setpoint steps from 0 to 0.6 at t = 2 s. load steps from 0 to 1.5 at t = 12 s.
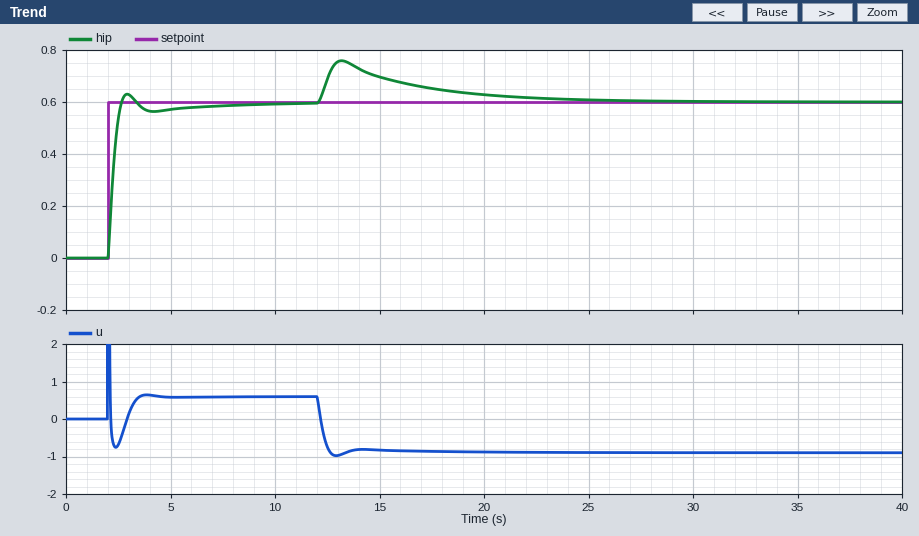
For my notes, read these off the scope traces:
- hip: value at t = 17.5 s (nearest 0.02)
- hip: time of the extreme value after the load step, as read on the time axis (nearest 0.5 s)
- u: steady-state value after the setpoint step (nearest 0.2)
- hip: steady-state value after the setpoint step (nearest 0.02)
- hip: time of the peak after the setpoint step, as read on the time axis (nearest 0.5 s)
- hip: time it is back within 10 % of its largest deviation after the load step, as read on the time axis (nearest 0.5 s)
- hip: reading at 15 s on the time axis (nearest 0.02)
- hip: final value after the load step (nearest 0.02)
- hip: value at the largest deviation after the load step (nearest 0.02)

0.66
13.0 s
0.6
0.60
3.0 s
22.0 s
0.70
0.60
0.76
